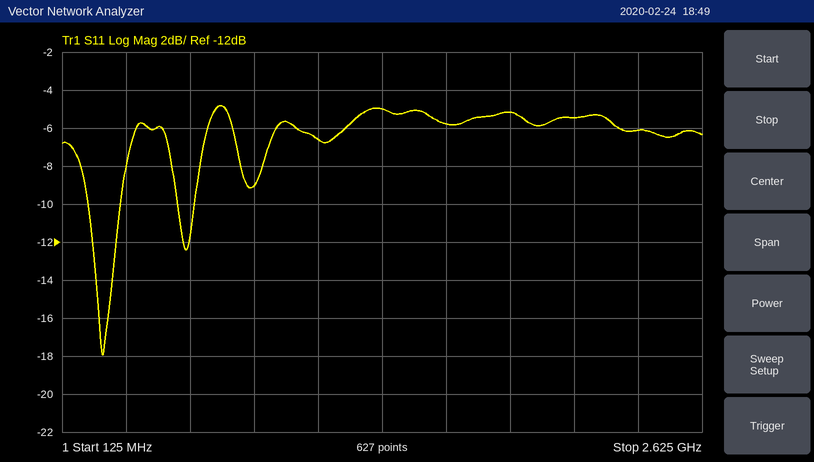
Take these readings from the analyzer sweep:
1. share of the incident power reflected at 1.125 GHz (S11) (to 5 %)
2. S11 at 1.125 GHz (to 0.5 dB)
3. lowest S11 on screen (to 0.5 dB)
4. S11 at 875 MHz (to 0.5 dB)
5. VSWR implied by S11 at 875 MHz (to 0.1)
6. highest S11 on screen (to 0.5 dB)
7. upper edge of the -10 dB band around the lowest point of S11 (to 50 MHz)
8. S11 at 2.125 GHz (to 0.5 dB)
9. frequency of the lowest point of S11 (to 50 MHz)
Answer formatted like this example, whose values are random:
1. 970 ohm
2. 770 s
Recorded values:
1. 20 %
2. -6.5 dB
3. -18.0 dB
4. -9.0 dB
5. 2.1
6. -5.0 dB
7. 350 MHz
8. -5.5 dB
9. 300 MHz
